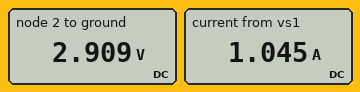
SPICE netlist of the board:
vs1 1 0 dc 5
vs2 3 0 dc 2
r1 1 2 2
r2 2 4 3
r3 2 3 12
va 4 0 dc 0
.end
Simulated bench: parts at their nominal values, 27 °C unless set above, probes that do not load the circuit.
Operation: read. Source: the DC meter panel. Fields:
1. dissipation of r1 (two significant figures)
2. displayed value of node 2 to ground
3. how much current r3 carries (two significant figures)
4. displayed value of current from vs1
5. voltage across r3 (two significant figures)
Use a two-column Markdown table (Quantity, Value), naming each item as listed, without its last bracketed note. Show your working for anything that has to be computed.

| Quantity | Value |
|---|---|
| dissipation of r1 | (5 V - 2.909 V)^2 / 2 Ω = 2.2 W |
| displayed value of node 2 to ground | 2.909 V |
| how much current r3 carries | (2.909 V - 2 V) / 12 Ω = 76 mA |
| displayed value of current from vs1 | 1.045 A |
| voltage across r3 | 2.909 V - 2 V = 910 mV |
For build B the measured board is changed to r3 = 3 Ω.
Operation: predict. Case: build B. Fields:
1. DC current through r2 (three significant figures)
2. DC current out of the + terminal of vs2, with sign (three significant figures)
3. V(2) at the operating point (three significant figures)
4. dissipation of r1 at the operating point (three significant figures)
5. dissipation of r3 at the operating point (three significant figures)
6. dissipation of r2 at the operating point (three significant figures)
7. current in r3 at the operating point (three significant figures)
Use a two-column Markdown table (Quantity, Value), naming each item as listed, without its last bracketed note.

| Quantity | Value |
|---|---|
| DC current through r2 | 905 mA |
| DC current out of the + terminal of vs2, with sign | -238 mA |
| V(2) at the operating point | 2.71 V |
| dissipation of r1 at the operating point | 2.61 W |
| dissipation of r3 at the operating point | 170 mW |
| dissipation of r2 at the operating point | 2.46 W |
| current in r3 at the operating point | 238 mA |
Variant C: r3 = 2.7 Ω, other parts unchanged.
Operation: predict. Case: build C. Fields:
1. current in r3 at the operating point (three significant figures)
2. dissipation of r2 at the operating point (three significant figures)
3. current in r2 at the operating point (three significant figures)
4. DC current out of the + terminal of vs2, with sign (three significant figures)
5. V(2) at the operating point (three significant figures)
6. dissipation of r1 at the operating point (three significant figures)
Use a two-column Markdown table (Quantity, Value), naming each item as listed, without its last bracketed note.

| Quantity | Value |
|---|---|
| current in r3 at the operating point | 256 mA |
| dissipation of r2 at the operating point | 2.42 W |
| current in r2 at the operating point | 897 mA |
| DC current out of the + terminal of vs2, with sign | -256 mA |
| V(2) at the operating point | 2.69 V |
| dissipation of r1 at the operating point | 2.66 W |
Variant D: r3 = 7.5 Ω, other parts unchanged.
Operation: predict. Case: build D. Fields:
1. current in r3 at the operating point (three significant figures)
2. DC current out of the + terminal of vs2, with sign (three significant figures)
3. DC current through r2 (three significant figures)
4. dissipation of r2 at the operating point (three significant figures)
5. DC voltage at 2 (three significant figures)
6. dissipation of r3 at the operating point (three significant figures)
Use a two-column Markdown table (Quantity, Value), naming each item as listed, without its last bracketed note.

| Quantity | Value |
|---|---|
| current in r3 at the operating point | 115 mA |
| DC current out of the + terminal of vs2, with sign | -115 mA |
| DC current through r2 | 954 mA |
| dissipation of r2 at the operating point | 2.73 W |
| DC voltage at 2 | 2.86 V |
| dissipation of r3 at the operating point | 99.1 mW |
